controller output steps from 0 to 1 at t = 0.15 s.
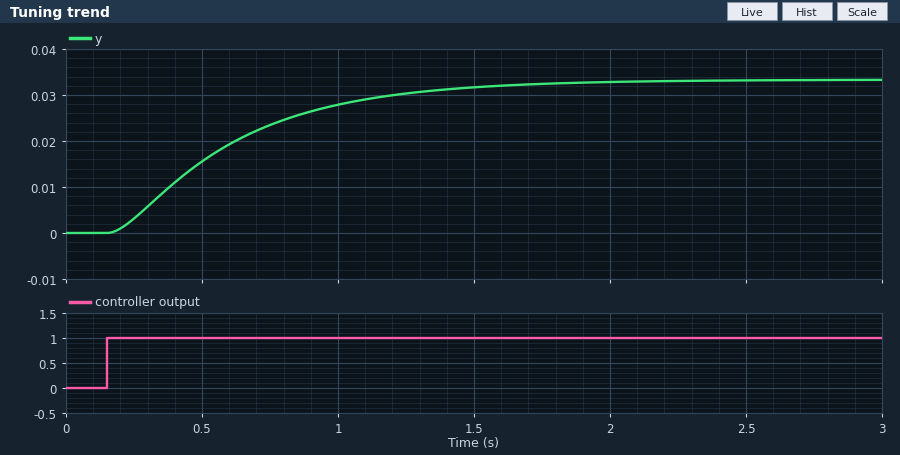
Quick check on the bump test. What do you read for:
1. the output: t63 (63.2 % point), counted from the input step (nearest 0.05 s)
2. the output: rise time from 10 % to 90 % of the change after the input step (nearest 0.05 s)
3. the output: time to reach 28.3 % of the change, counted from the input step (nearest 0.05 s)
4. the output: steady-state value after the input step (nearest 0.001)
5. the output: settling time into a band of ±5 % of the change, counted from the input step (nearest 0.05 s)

0.50 s
0.95 s
0.20 s
0.033
1.35 s
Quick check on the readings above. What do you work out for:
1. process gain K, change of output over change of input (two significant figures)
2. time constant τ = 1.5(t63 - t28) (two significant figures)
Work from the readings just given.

0.033
0.45 s
